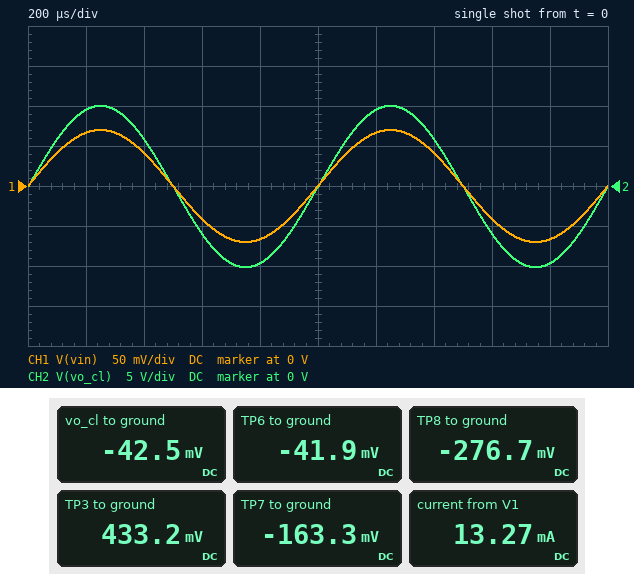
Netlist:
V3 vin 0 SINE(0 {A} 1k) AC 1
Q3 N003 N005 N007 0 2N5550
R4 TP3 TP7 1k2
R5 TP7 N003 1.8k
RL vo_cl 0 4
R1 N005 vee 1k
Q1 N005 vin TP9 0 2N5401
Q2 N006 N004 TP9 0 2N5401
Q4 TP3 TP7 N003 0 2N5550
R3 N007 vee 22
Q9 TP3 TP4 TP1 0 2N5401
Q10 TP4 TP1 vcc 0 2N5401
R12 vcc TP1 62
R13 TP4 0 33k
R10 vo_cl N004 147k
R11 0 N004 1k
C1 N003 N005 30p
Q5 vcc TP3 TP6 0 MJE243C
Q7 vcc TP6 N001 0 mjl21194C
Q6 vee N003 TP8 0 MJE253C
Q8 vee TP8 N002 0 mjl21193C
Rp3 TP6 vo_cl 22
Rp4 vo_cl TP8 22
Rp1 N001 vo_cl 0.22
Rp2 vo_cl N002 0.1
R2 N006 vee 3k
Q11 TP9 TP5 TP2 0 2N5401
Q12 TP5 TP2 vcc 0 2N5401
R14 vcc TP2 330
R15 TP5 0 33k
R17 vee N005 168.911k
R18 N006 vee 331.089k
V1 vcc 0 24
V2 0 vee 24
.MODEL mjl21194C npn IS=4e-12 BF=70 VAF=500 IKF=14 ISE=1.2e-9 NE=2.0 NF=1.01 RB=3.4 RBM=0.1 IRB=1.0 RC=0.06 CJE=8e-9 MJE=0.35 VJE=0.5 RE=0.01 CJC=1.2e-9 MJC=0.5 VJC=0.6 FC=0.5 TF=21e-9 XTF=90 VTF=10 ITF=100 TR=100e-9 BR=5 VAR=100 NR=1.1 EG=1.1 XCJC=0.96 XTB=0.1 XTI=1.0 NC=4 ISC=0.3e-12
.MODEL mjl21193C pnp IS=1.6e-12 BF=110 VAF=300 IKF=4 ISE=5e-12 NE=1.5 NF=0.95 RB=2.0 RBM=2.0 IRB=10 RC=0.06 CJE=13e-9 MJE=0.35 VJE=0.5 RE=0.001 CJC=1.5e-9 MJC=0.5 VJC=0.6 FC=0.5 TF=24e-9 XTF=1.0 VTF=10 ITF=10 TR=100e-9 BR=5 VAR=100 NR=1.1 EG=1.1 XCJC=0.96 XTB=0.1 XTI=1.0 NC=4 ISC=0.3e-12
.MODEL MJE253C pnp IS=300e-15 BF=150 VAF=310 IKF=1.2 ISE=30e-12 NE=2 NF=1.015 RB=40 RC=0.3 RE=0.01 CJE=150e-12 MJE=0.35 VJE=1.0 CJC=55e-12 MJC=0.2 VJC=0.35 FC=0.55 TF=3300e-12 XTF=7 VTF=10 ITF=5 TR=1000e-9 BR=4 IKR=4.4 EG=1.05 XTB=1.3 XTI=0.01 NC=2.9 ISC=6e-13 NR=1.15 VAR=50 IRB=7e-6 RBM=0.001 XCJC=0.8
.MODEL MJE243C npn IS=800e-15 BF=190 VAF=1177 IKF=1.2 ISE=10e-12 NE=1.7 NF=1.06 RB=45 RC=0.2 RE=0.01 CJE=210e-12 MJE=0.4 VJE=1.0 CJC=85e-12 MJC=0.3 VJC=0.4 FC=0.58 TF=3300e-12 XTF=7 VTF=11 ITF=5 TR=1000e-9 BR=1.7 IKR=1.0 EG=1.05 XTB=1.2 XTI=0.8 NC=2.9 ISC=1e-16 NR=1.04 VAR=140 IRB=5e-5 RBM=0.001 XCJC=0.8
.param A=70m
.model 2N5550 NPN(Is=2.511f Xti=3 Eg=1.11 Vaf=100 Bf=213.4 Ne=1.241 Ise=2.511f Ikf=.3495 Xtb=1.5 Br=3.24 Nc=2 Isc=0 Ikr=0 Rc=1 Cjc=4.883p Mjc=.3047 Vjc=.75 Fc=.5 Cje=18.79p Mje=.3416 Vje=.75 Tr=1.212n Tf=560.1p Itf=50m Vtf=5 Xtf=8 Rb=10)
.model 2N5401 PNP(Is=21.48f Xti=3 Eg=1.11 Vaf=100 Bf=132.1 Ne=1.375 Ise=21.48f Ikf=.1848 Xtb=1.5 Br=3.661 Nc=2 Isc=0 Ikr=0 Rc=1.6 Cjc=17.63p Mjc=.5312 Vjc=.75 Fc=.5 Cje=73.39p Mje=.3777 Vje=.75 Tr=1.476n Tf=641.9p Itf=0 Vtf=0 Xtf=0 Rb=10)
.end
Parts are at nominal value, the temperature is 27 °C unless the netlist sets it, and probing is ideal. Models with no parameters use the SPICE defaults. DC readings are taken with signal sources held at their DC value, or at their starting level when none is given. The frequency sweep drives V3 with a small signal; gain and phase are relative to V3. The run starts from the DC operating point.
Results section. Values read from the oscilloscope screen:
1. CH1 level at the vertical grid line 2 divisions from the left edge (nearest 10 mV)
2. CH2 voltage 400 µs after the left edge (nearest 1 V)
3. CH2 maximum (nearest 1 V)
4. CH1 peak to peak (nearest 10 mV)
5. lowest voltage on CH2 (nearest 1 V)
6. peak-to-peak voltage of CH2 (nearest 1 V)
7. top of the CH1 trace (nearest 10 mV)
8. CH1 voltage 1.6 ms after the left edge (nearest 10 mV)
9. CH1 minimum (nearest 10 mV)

40 mV
6 V
10 V
140 mV
-10 V
20 V
70 mV
-40 mV
-70 mV
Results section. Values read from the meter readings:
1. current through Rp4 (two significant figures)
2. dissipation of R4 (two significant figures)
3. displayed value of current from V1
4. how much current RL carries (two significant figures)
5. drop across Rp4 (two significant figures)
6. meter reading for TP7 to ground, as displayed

11 mA
300 µW
13.27 mA
11 mA
230 mV
-163.3 mV
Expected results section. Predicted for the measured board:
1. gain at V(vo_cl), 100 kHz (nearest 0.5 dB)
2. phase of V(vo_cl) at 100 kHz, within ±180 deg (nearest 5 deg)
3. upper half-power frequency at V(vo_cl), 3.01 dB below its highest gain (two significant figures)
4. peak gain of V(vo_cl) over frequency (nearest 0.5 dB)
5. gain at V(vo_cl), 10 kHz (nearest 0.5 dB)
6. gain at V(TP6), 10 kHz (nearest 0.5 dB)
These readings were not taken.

35.5 dB
-50 deg
79 kHz
39.5 dB
39.5 dB
40.5 dB
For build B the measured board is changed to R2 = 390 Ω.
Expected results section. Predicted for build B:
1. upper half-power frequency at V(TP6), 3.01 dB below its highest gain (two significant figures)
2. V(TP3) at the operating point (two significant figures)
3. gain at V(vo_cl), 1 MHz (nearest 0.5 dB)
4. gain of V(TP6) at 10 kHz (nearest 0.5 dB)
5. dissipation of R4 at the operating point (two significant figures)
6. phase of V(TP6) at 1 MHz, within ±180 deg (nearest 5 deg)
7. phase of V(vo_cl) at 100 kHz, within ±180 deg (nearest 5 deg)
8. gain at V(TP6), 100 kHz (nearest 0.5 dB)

120 kHz
720 mV
23.0 dB
51.5 dB
300 µW
-130 deg
-40 deg
49.5 dB
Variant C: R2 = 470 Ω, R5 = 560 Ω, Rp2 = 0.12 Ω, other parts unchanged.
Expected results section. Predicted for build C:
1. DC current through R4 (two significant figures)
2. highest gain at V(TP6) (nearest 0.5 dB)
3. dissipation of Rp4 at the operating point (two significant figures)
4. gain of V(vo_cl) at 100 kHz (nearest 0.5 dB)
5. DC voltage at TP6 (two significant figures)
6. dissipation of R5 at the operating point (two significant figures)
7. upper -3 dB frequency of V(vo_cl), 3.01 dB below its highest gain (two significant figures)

1.4 mA
45.5 dB
13 mW
42.5 dB
580 mV
1.0 mW
430 kHz
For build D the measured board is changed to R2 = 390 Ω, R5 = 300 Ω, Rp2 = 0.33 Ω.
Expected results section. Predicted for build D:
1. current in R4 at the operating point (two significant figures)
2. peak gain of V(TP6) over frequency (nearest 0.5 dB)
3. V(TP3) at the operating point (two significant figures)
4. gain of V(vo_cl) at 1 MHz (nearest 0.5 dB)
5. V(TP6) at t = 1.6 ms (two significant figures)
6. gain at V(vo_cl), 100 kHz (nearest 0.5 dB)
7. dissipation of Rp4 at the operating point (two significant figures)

2.5 mA
43.5 dB
1.9 V
37.0 dB
-5.0 V
43.0 dB
70 mW
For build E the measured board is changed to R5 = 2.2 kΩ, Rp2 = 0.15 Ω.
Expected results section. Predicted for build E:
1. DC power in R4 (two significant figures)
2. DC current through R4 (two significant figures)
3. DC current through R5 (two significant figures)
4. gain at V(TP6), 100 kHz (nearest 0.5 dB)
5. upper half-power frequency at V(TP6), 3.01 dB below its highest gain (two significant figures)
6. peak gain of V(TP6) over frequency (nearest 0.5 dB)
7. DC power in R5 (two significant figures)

210 µW
420 µA
340 µA
35.5 dB
77 kHz
39.5 dB
260 µW
